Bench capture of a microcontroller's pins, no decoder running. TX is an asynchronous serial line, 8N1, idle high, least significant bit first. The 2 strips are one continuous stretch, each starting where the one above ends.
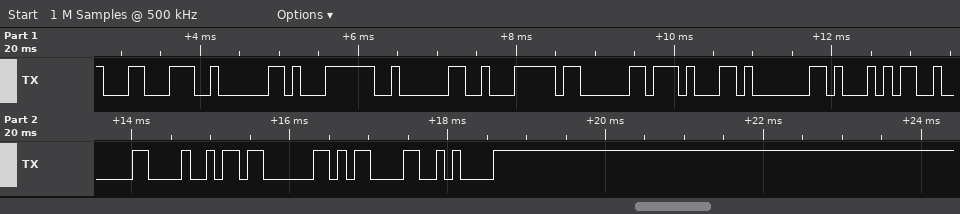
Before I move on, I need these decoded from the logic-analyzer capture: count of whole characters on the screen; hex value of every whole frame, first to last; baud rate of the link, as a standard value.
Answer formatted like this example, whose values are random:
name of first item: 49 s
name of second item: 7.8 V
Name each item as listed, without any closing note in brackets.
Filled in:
count of whole characters on the screen: 14
hex value of every whole frame, first to last: 0x8C 0x02 0xF1 0x02 0xE2 0x03 0x17 0x01 0x51 0x02 0x48 0x03 0x0D 0x0A
baud rate of the link, as a standard value: 9600 baud
